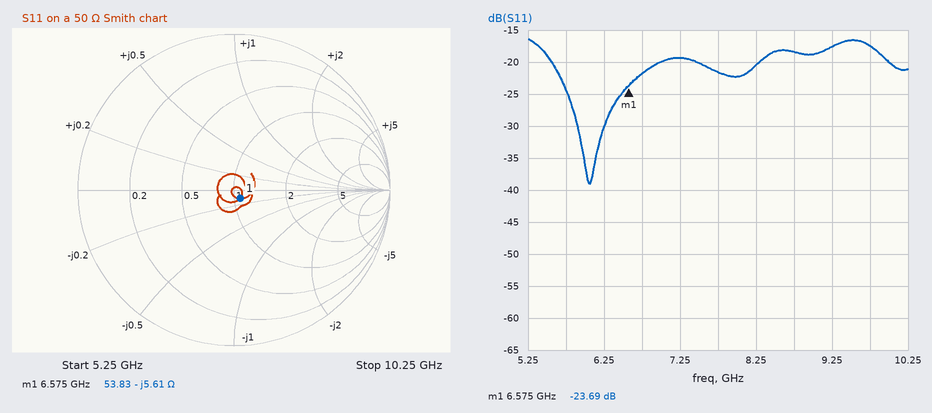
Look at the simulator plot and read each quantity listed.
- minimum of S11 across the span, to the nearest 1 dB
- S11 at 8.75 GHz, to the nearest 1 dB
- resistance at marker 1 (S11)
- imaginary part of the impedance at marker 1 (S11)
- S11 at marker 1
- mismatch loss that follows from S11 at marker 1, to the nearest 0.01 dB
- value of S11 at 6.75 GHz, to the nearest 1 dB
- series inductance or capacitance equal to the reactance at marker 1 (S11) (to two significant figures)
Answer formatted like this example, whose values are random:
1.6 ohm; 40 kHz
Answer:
-39 dB; -18 dB; 53.83 Ω; -5.61 Ω; -23.69 dB; 0.02 dB; -22 dB; 4.3 pF
